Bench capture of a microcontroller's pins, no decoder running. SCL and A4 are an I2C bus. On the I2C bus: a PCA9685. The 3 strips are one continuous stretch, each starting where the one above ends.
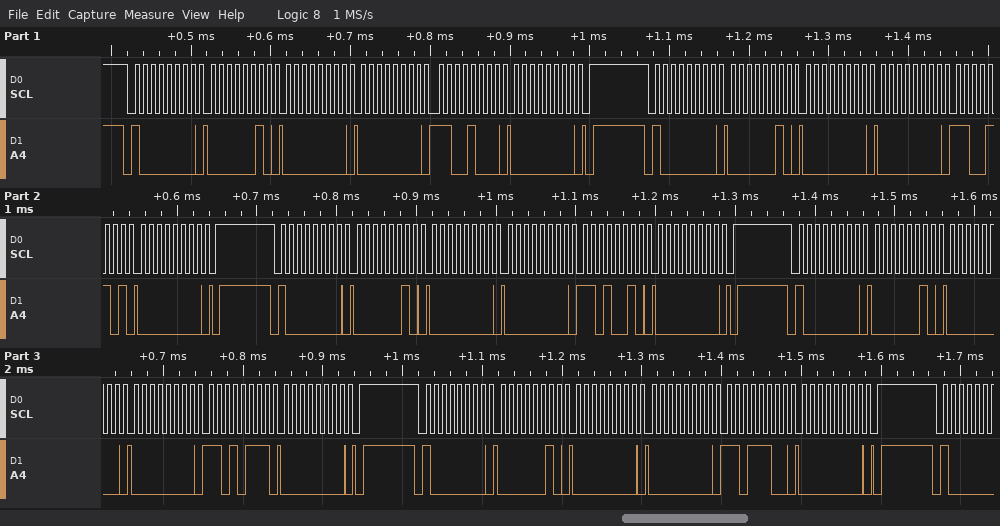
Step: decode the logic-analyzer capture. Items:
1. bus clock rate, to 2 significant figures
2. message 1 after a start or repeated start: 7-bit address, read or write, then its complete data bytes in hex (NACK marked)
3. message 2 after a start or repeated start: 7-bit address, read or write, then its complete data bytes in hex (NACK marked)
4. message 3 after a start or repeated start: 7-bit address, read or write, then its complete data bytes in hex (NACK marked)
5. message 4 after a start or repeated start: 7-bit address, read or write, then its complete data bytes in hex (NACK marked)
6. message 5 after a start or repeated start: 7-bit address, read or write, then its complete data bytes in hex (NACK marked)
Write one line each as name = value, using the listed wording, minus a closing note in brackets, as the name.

bus clock rate, to 2 significant figures = 100 kHz
message 1 after a start or repeated start: 7-bit address, read or write, then its complete data bytes in hex = 0x40 write: 02 00 00 C8 00
message 2 after a start or repeated start: 7-bit address, read or write, then its complete data bytes in hex = 0x40 write: 02 00 00 CD 00
message 3 after a start or repeated start: 7-bit address, read or write, then its complete data bytes in hex = 0x40 write: 02 00 00 D2 00
message 4 after a start or repeated start: 7-bit address, read or write, then its complete data bytes in hex = 0x40 write: 02 00 00 D7 00
message 5 after a start or repeated start: 7-bit address, read or write, then its complete data bytes in hex = 0x40 write: 02 00 00 DC 00
